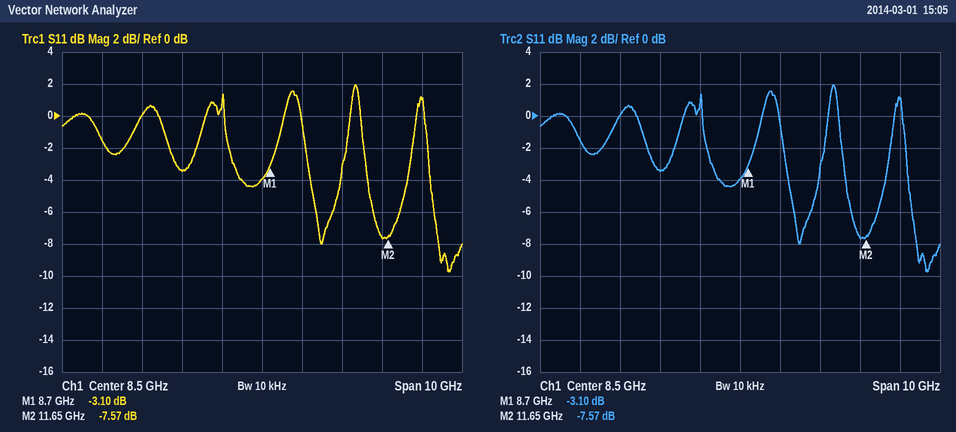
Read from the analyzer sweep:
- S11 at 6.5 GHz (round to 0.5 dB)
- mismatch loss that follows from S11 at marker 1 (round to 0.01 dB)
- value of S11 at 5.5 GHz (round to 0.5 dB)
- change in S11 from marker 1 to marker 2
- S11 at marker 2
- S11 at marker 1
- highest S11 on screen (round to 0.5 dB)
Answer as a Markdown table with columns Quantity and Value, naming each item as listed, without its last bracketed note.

| Quantity | Value |
|---|---|
| S11 at 6.5 GHz | -3.5 dB |
| mismatch loss that follows from S11 at marker 1 | 2.92 dB |
| value of S11 at 5.5 GHz | 0.0 dB |
| change in S11 from marker 1 to marker 2 | -4.47 dB |
| S11 at marker 2 | -7.57 dB |
| S11 at marker 1 | -3.10 dB |
| highest S11 on screen | 2.0 dB |
